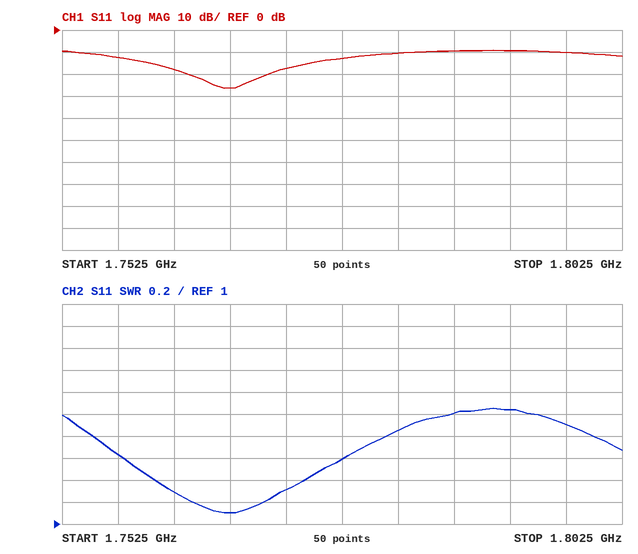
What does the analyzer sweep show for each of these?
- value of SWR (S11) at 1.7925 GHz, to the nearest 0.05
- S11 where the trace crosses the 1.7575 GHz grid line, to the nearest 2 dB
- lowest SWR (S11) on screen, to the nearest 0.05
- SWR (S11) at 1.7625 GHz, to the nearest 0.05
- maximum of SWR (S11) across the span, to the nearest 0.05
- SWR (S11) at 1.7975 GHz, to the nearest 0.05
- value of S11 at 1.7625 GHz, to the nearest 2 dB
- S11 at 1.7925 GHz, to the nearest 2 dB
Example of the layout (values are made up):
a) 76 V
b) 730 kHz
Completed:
a) 2.05
b) -12 dB
c) 1.10
d) 1.30
e) 2.05
f) 1.90
g) -18 dB
h) -10 dB
